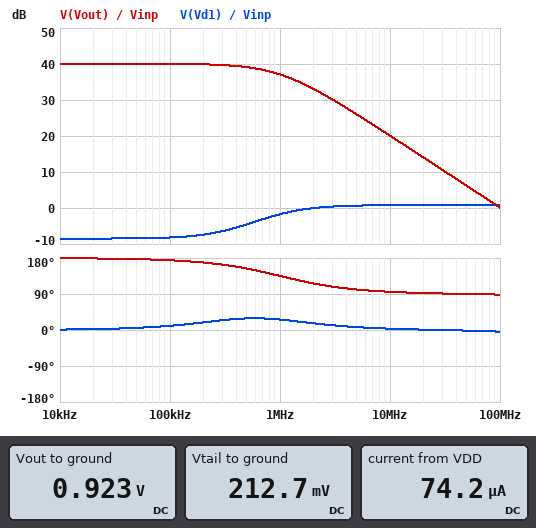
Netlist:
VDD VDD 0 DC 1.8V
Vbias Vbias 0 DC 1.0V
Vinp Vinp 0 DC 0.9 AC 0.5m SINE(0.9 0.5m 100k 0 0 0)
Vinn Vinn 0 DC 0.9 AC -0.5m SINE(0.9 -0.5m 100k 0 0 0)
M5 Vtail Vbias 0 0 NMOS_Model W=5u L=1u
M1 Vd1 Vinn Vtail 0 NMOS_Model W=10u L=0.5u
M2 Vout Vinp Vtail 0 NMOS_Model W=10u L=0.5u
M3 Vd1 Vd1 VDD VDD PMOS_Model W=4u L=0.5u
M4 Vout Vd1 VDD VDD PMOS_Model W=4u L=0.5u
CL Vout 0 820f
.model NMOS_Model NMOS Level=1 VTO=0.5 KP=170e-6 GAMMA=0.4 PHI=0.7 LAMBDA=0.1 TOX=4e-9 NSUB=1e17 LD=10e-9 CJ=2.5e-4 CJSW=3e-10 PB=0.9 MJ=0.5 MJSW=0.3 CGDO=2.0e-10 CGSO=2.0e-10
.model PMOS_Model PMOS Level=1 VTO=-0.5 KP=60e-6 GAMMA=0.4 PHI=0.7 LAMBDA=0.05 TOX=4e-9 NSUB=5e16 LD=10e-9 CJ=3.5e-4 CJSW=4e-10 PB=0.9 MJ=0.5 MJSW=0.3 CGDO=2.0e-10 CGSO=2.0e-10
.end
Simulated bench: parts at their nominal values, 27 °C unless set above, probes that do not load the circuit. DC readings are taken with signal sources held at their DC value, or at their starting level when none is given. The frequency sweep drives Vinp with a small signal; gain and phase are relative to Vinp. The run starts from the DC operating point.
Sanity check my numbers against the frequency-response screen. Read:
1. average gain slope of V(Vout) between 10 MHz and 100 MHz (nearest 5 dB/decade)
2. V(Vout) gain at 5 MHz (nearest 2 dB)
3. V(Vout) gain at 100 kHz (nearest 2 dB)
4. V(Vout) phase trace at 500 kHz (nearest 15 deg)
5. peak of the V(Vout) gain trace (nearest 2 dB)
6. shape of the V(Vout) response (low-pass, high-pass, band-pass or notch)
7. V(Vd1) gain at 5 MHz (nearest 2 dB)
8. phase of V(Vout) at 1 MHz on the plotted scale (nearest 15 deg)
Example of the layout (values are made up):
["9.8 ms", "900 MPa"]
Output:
["-20 dB/decade", "26 dB", "40 dB", "150 deg", "40 dB", "low-pass", "0 dB", "135 deg"]
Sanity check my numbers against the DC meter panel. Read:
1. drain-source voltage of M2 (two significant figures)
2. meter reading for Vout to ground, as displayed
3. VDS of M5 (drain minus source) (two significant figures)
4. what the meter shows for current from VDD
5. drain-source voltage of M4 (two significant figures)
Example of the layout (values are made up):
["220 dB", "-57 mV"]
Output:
["710 mV", "0.923 V", "210 mV", "74.2 µA", "-880 mV"]
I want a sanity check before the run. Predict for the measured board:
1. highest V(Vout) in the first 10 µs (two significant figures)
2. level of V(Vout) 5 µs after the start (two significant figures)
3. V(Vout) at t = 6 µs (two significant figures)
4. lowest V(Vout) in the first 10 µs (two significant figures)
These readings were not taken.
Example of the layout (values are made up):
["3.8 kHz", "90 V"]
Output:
["1.0 V", "910 mV", "970 mV", "820 mV"]
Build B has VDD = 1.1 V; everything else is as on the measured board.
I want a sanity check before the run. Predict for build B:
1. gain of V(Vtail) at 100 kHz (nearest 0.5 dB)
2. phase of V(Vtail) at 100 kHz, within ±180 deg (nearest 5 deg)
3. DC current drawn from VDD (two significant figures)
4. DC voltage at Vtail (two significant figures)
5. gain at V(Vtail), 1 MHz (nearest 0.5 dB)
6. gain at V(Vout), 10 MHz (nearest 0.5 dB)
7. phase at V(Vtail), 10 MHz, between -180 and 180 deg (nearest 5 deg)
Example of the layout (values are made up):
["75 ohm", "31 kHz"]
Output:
["-58.5 dB", "20 deg", "66 µA", "180 mV", "-47.0 dB", "-5.5 dB", "75 deg"]
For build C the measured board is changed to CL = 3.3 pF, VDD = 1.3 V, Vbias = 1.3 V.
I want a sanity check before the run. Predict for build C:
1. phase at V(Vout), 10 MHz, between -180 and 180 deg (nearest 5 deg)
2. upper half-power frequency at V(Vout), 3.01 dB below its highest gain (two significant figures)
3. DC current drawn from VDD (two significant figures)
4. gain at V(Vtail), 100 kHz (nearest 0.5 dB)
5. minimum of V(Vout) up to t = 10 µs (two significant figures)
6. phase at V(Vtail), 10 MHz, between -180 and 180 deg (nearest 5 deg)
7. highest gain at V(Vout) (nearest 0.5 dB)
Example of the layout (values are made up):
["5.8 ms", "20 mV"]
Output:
["110 deg", "4.0 MHz", "110 µA", "-38.5 dB", "330 mV", "20 deg", "15.5 dB"]
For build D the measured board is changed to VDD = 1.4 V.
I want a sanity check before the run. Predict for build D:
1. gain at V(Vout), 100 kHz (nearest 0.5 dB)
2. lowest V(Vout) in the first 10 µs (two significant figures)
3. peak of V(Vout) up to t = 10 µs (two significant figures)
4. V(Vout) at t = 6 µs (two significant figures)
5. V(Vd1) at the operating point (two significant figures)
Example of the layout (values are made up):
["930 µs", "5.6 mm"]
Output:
["39.5 dB", "430 mV", "620 mV", "570 mV", "520 mV"]
